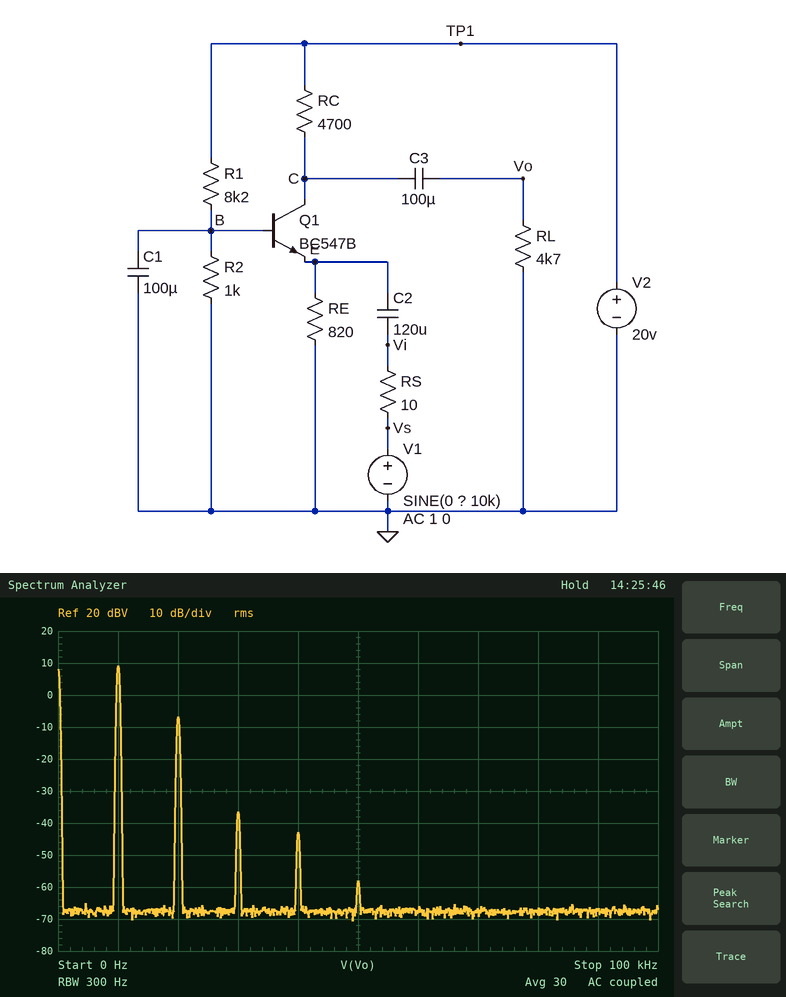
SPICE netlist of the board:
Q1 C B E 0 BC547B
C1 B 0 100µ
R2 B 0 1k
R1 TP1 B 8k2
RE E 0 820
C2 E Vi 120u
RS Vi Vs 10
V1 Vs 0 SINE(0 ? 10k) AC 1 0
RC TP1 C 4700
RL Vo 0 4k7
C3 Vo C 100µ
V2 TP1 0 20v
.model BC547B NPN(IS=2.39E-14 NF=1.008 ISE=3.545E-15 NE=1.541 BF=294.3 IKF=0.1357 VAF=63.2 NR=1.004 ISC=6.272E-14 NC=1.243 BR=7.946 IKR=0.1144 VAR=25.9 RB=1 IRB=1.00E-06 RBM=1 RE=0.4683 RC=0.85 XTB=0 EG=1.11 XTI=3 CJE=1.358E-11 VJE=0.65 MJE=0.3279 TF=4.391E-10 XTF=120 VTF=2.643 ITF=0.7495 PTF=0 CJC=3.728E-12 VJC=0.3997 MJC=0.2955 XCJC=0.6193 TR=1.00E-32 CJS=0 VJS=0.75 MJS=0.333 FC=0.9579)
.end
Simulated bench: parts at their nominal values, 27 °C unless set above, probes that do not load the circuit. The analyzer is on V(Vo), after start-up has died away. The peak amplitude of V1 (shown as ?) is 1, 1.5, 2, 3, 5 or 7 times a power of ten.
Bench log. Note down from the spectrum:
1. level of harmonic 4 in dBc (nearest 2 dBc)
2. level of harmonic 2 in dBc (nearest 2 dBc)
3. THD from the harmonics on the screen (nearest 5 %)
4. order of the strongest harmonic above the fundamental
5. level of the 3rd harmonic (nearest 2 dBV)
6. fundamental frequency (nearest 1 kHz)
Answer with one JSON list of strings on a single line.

["-52 dBc", "-16 dBc", "15 %", "2", "-36 dBV", "10 kHz"]
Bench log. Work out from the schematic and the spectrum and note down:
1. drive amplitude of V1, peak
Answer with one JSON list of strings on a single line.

["50 mV"]
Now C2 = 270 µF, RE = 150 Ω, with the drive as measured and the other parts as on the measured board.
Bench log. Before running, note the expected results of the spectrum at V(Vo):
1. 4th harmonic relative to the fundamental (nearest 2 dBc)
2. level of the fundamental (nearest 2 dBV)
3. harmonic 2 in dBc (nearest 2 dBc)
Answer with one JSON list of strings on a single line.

["-22 dBc", "-2 dBV", "-4 dBc"]
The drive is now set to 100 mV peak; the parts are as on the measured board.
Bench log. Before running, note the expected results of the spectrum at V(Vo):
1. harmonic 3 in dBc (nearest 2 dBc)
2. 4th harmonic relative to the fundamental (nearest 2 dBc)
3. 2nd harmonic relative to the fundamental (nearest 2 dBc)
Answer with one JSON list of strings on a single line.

["-34 dBc", "-34 dBc", "-10 dBc"]
